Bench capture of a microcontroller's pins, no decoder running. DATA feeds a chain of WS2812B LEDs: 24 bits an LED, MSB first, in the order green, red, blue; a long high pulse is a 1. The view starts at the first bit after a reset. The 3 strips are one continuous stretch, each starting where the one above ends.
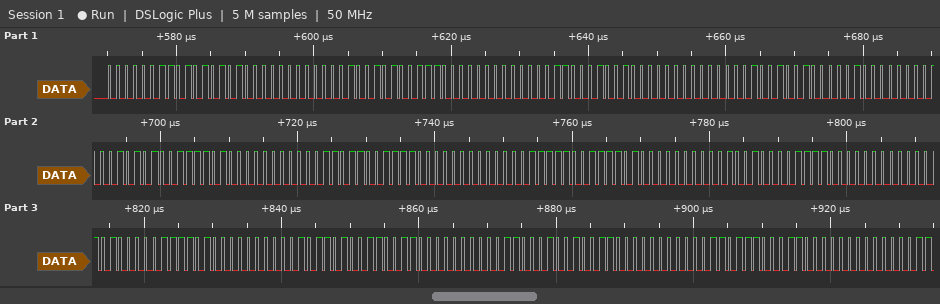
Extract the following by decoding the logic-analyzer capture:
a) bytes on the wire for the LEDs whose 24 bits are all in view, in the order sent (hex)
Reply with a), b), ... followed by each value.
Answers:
a) 03 55 00 09 4E 00 0C 48 00 12 41 00 15 3D 00 1B 3C 00 1F 3D 00 24 3C 00 28 3D 00 2D 33 00 31 26 00 37 18 00
